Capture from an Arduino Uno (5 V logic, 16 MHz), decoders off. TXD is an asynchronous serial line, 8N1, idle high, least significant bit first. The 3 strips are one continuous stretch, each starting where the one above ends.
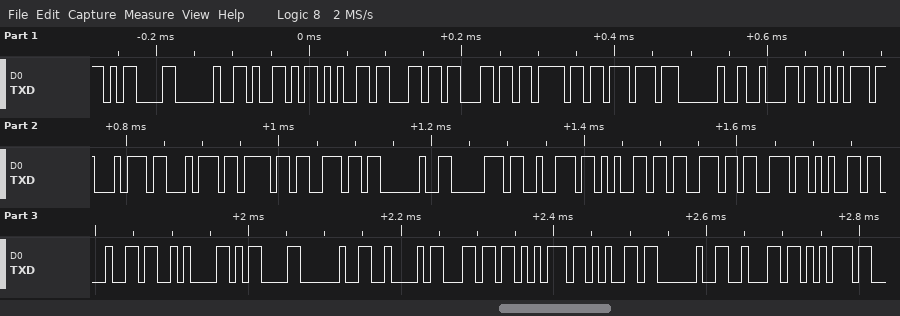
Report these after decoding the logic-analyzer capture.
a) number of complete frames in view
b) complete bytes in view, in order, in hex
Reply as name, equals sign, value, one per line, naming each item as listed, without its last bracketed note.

number of complete frames in view = 33
complete bytes in view, in order, in hex = 0x0D 0x20 0x59 0x65 0x6C 0x6C 0x6F 0x77 0x20 0x62 0x75 0x74 0x74 0x6F 0x6E 0x20 0x70 0x72 0x65 0x73 0x73 0x65 0x64 0x0A 0x0D 0x20 0x42 0x6C 0x75 0x65 0x20 0x62 0x75
